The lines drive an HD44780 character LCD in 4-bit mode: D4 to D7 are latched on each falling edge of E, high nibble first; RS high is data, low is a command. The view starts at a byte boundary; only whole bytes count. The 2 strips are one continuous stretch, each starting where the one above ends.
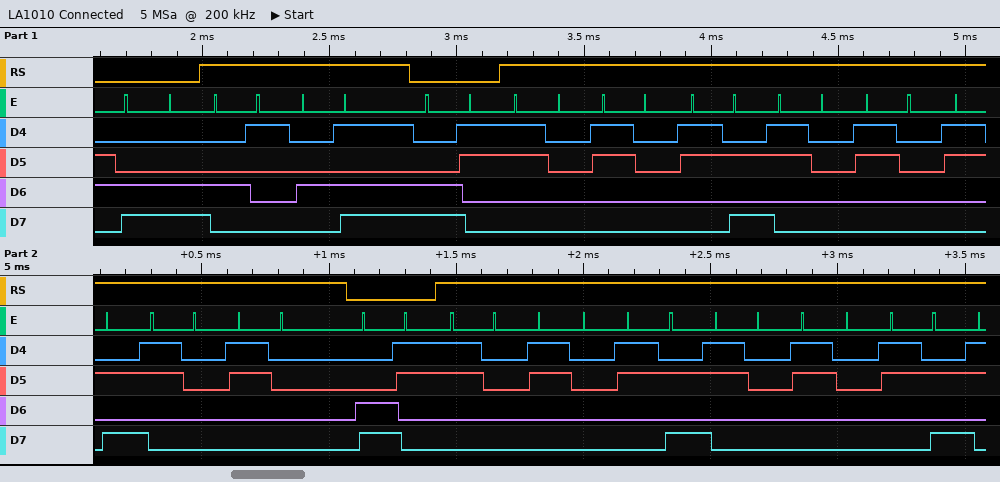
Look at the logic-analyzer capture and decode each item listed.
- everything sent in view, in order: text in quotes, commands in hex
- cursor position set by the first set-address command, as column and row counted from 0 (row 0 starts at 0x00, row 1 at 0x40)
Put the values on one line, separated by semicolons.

0xCC "AM" 0xC3 "00:00:00" 0xC3 "00:00:"; column 12, row 1
